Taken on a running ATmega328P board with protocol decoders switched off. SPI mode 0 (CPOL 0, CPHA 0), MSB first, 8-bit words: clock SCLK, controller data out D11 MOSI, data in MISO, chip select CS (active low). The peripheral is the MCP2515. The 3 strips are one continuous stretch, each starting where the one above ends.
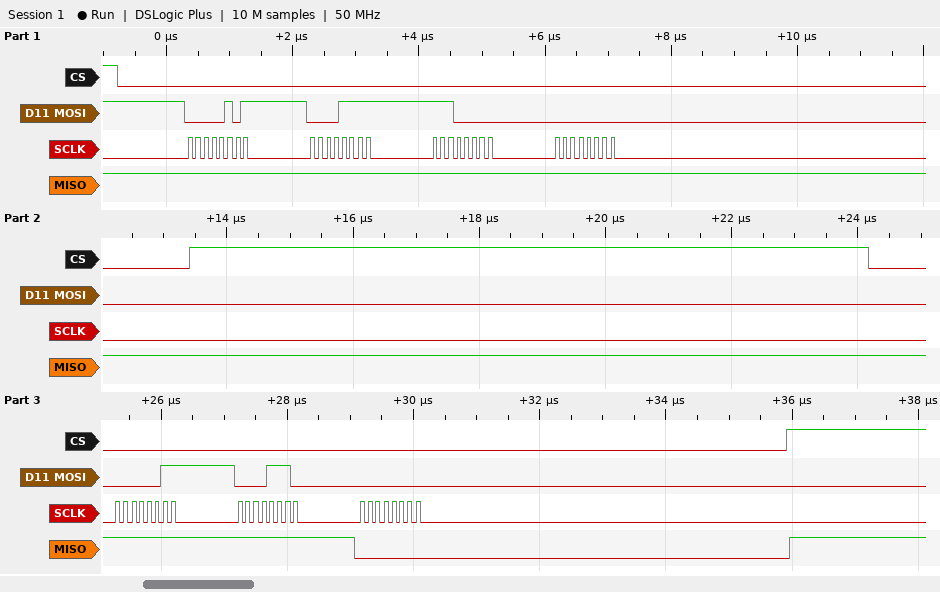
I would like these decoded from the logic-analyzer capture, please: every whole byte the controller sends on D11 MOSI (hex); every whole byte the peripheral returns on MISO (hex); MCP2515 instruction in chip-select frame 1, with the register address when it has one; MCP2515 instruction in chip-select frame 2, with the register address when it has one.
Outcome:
05 0F E0 00 03 0E 00
FF FF FF FF FF FF 00
BIT MODIFY 0x0F
READ 0x0E
